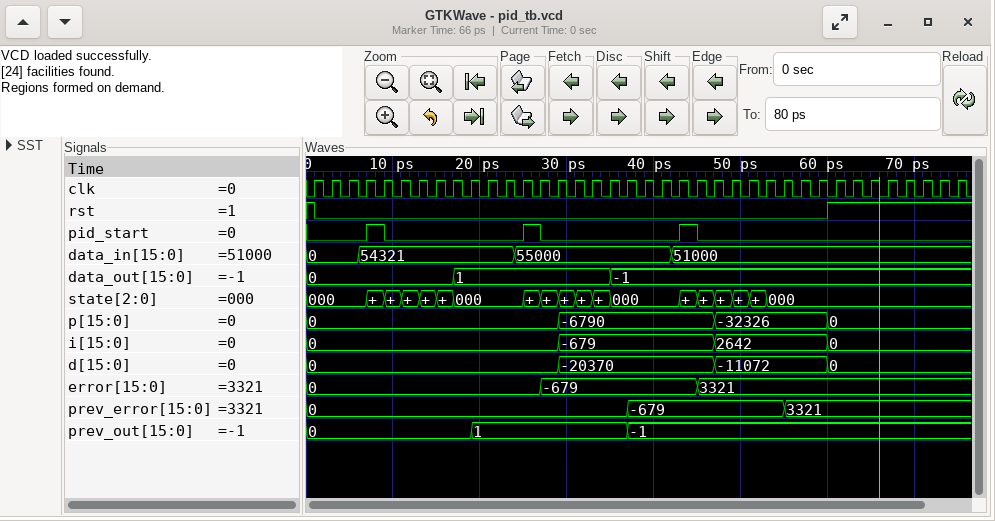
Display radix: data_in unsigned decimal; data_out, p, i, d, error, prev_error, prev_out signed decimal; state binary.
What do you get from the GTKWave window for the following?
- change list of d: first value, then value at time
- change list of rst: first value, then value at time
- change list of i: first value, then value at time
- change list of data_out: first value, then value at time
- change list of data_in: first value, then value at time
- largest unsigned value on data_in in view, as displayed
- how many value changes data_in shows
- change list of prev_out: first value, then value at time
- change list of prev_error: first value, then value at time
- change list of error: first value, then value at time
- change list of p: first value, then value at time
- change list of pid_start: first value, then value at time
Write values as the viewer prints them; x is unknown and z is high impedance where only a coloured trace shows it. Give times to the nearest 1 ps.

0, -20370 at 29 ps, -11072 at 47 ps, 0 at 60 ps
1, 0 at 1 ps, 1 at 60 ps
0, -679 at 29 ps, 2642 at 47 ps, 0 at 60 ps
0, 1 at 17 ps, -1 at 35 ps
0, 54321 at 6 ps, 55000 at 24 ps, 51000 at 42 ps
55000
3
0, 1 at 19 ps, -1 at 37 ps
0, -679 at 37 ps, 3321 at 55 ps
0, -679 at 27 ps, 3321 at 45 ps
0, -6790 at 29 ps, -32326 at 47 ps, 0 at 60 ps
0, 1 at 7 ps, 0 at 9 ps, 1 at 25 ps, 0 at 27 ps, 1 at 43 ps, 0 at 45 ps
